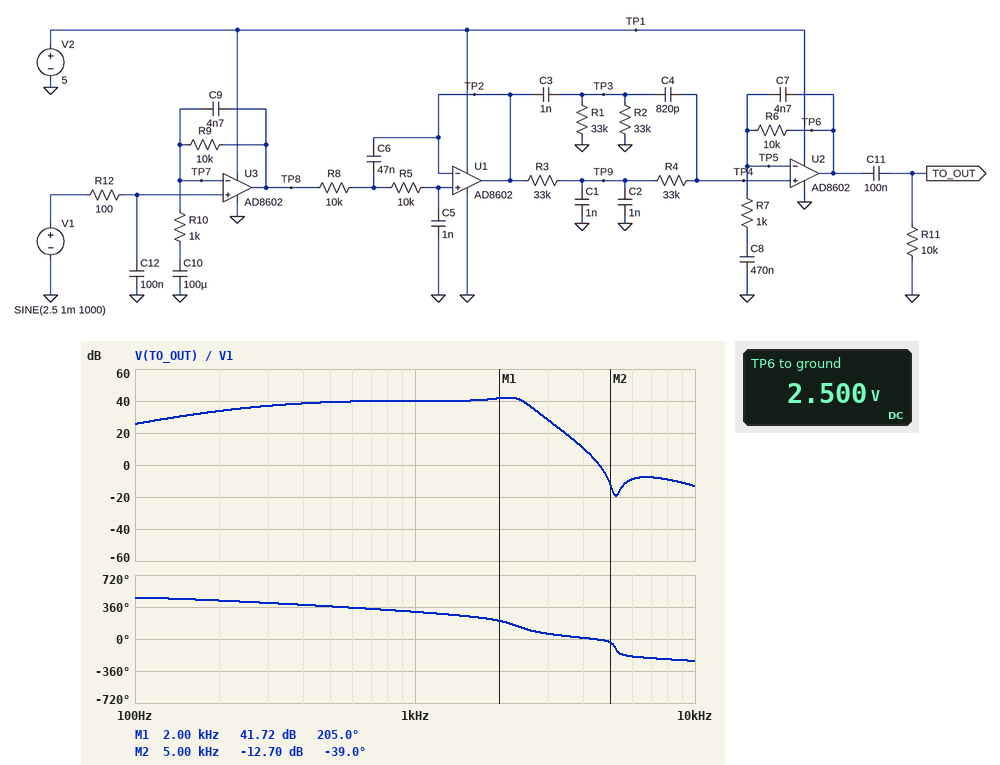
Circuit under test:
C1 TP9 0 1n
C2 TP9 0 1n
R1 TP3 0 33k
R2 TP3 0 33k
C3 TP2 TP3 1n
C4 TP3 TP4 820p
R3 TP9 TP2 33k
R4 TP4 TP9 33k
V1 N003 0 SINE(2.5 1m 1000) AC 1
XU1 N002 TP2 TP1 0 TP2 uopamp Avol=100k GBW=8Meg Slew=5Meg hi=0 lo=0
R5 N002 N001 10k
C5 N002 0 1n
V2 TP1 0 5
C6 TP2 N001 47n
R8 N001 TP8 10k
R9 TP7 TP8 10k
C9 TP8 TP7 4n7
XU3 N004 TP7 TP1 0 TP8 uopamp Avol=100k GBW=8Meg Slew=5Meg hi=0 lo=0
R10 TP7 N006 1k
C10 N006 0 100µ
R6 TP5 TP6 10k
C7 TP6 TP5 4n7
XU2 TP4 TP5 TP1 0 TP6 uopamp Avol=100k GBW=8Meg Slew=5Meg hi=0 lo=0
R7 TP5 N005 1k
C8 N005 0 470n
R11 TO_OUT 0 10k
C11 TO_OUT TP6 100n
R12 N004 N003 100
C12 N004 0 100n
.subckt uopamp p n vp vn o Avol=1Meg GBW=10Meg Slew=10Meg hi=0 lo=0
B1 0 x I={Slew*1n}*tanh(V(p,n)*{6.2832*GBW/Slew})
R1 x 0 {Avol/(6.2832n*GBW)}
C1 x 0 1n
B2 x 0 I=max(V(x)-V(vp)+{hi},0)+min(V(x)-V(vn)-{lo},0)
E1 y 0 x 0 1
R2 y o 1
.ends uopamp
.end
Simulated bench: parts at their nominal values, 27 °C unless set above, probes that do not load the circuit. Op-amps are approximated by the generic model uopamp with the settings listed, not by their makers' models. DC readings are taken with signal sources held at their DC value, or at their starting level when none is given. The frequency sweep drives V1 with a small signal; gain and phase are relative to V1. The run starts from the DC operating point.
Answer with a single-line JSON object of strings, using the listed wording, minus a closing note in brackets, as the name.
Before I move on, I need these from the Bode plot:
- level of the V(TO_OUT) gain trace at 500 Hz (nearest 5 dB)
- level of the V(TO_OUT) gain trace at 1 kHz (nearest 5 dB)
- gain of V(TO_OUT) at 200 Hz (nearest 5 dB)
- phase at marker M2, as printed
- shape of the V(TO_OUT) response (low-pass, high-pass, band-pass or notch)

{"level of the V(TO_OUT) gain trace at 500 Hz": "40 dB", "level of the V(TO_OUT) gain trace at 1 kHz": "40 dB", "gain of V(TO_OUT) at 200 Hz": "35 dB", "phase at marker M2, as printed": "-39.0 deg", "shape of the V(TO_OUT) response": "band-pass"}
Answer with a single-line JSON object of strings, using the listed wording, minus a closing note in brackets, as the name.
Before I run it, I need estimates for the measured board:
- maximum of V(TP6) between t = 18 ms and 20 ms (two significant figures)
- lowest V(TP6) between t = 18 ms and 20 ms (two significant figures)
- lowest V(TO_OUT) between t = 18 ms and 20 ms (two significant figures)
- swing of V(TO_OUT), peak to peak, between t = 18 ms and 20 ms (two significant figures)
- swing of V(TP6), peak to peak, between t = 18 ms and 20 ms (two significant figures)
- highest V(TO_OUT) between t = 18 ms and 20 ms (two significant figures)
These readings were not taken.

{"maximum of V(TP6) between t = 18 ms and 20 ms": "2.6 V", "lowest V(TP6) between t = 18 ms and 20 ms": "2.4 V", "lowest V(TO_OUT) between t = 18 ms and 20 ms": "-100 mV", "swing of V(TO_OUT), peak to peak, between t = 18 ms and 20 ms": "200 mV", "swing of V(TP6), peak to peak, between t = 18 ms and 20 ms": "200 mV", "highest V(TO_OUT) between t = 18 ms and 20 ms": "100 mV"}
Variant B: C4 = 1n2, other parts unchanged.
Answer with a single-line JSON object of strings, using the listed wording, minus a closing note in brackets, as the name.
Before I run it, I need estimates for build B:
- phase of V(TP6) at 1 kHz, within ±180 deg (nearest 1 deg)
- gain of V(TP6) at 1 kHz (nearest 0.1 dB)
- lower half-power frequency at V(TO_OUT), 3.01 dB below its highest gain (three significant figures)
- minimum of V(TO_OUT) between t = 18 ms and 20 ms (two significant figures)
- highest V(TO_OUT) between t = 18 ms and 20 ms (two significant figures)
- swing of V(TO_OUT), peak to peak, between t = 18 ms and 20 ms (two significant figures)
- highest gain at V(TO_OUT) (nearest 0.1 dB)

{"phase of V(TP6) at 1 kHz, within ±180 deg": "-69 deg", "gain of V(TP6) at 1 kHz": "39.3 dB", "lower half-power frequency at V(TO_OUT), 3.01 dB below its highest gain": "311 Hz", "minimum of V(TO_OUT) between t = 18 ms and 20 ms": "-91 mV", "highest V(TO_OUT) between t = 18 ms and 20 ms": "91 mV", "swing of V(TO_OUT), peak to peak, between t = 18 ms and 20 ms": "180 mV", "highest gain at V(TO_OUT)": "40.1 dB"}
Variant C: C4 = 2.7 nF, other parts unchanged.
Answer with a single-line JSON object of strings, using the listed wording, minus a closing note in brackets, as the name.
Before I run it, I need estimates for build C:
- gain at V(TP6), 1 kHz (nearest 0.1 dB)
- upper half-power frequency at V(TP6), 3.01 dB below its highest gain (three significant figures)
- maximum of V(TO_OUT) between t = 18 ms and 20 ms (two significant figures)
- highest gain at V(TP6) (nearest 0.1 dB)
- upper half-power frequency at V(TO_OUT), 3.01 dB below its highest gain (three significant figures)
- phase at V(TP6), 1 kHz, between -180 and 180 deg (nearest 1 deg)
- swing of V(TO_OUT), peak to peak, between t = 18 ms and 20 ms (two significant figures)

{"gain at V(TP6), 1 kHz": "36.0 dB", "upper half-power frequency at V(TP6), 3.01 dB below its highest gain": "1.24 kHz", "maximum of V(TO_OUT) between t = 18 ms and 20 ms": "62 mV", "highest gain at V(TP6)": "38.0 dB", "upper half-power frequency at V(TO_OUT), 3.01 dB below its highest gain": "1.35 kHz", "phase at V(TP6), 1 kHz, between -180 and 180 deg": "-79 deg", "swing of V(TO_OUT), peak to peak, between t = 18 ms and 20 ms": "120 mV"}
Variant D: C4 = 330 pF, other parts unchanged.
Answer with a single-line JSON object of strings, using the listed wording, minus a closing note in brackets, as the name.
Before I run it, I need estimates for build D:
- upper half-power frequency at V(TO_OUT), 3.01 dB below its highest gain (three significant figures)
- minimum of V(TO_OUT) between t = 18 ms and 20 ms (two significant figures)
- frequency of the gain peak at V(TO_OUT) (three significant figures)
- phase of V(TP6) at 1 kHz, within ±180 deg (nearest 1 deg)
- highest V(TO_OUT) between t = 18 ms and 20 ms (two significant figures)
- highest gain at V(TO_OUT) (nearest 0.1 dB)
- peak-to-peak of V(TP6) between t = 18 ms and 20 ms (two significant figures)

{"upper half-power frequency at V(TO_OUT), 3.01 dB below its highest gain": "2.49 kHz", "minimum of V(TO_OUT) between t = 18 ms and 20 ms": "-110 mV", "frequency of the gain peak at V(TO_OUT)": "2.19 kHz", "phase of V(TP6) at 1 kHz, within ±180 deg": "-55 deg", "highest V(TO_OUT) between t = 18 ms and 20 ms": "110 mV", "highest gain at V(TO_OUT)": "44.9 dB", "peak-to-peak of V(TP6) between t = 18 ms and 20 ms": "230 mV"}
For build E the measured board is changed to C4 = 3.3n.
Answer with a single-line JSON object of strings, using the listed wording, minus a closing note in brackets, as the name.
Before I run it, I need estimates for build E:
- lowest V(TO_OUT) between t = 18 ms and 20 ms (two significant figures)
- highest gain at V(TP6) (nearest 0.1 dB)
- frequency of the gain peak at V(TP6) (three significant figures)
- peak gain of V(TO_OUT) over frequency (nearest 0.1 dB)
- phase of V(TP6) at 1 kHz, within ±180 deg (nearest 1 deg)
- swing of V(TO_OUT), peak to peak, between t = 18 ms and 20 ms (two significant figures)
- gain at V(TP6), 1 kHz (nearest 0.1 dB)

{"lowest V(TO_OUT) between t = 18 ms and 20 ms": "-54 mV", "highest gain at V(TP6)": "37.4 dB", "frequency of the gain peak at V(TP6)": "421 Hz", "peak gain of V(TO_OUT) over frequency": "36.9 dB", "phase of V(TP6) at 1 kHz, within ±180 deg": "-79 deg", "swing of V(TO_OUT), peak to peak, between t = 18 ms and 20 ms": "110 mV", "gain at V(TP6), 1 kHz": "34.8 dB"}
